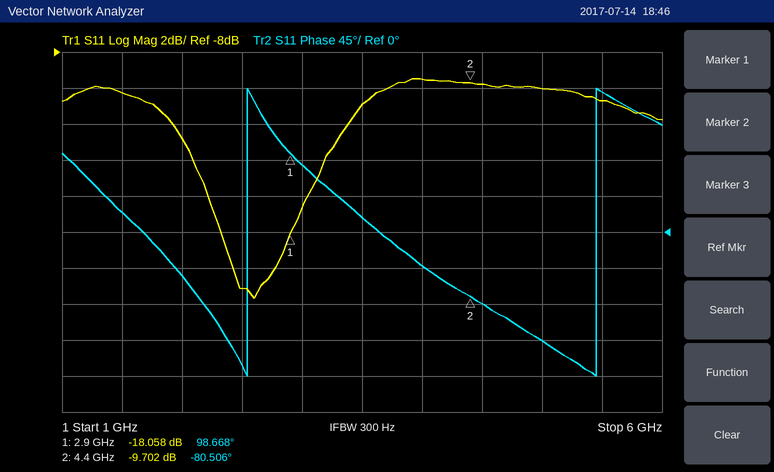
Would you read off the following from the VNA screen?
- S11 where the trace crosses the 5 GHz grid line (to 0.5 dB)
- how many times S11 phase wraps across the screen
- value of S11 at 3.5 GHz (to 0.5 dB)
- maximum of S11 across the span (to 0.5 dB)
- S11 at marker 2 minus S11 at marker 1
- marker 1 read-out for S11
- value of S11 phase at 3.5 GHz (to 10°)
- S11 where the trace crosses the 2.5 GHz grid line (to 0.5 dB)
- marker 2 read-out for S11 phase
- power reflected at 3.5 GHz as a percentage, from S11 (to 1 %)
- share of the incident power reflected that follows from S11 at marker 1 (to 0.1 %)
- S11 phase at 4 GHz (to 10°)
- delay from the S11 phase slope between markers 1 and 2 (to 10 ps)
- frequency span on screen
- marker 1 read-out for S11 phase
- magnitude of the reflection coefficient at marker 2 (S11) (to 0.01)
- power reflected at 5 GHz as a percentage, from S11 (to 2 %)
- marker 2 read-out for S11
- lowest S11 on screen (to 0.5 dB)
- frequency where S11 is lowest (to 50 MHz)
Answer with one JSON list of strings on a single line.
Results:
["-10.0 dB", "2", "-11.0 dB", "-9.5 dB", "8.356 dB", "-18.058 dB", "20°", "-21.0 dB", "-80.506°", "8 %", "1.6 %", "-40°", "330 ps", "5 GHz", "98.668°", "0.33", "10 %", "-9.702 dB", "-21.5 dB", "2.60 GHz"]
